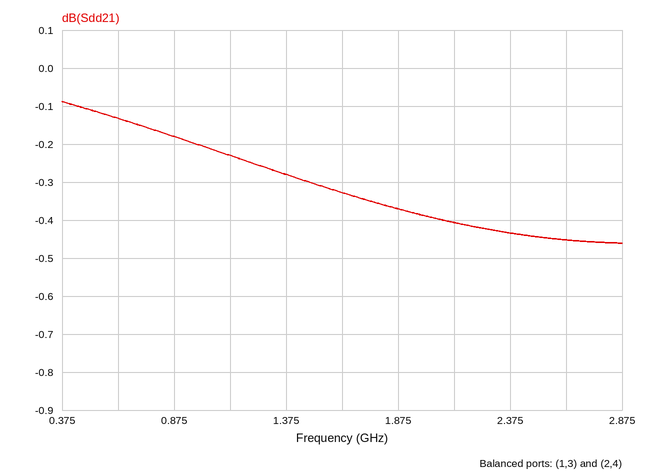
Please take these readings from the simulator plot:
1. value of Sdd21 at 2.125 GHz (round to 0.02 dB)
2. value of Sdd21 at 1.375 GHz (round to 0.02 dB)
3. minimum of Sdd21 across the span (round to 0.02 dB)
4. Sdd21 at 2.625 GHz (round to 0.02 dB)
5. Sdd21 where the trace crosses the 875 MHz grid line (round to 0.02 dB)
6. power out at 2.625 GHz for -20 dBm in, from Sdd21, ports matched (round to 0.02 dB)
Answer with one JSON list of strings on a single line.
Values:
["-0.40 dB", "-0.28 dB", "-0.46 dB", "-0.46 dB", "-0.18 dB", "-20.46 dBm"]
